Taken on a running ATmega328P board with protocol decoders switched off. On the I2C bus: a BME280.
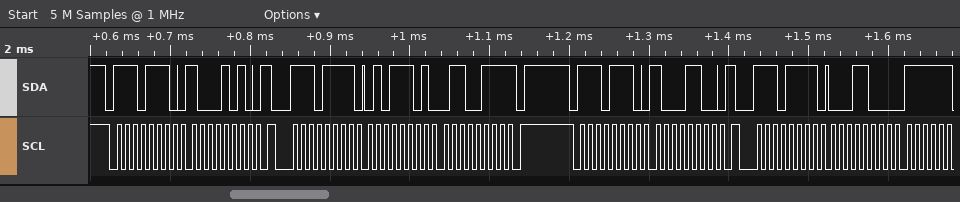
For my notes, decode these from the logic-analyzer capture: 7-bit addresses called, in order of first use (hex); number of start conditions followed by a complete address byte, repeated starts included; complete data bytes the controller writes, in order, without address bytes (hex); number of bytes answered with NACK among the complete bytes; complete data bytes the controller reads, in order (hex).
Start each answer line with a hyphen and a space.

- 0x77
- 4
- 8A 8C
- 1
- 5D 67 18
